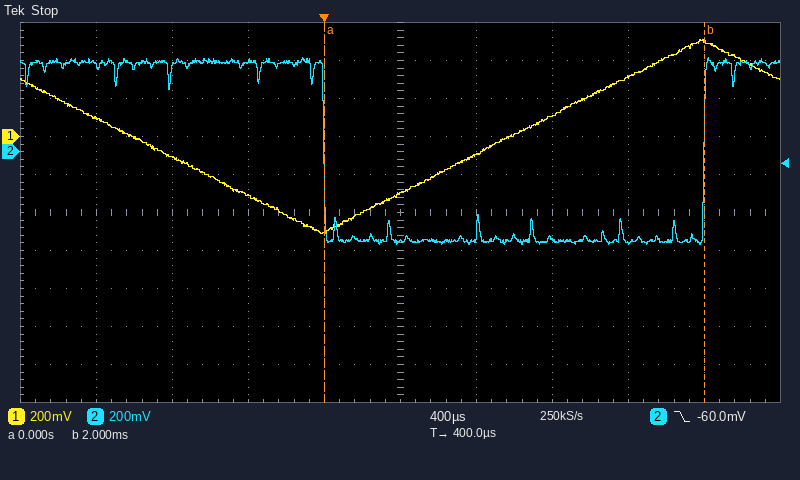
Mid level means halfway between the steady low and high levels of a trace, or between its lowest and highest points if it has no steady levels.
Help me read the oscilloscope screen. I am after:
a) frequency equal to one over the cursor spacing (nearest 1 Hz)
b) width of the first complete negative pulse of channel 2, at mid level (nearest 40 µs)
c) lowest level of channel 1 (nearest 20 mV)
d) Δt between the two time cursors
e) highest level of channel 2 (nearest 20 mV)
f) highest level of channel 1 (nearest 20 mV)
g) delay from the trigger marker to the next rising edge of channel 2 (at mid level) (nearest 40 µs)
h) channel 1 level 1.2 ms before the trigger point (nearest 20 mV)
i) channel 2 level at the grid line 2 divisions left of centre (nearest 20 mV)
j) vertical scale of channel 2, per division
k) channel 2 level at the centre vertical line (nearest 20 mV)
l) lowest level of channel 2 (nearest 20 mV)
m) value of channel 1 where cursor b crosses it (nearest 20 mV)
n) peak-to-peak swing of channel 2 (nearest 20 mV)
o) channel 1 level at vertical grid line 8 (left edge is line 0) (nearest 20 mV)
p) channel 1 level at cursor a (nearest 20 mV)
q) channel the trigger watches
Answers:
500 Hz
2.00 ms
-520 mV
2.00 ms
500 mV
520 mV
2.00 ms
100 mV
480 mV
200 mV
-480 mV
-480 mV
500 mV
980 mV
320 mV
-500 mV
channel 2
